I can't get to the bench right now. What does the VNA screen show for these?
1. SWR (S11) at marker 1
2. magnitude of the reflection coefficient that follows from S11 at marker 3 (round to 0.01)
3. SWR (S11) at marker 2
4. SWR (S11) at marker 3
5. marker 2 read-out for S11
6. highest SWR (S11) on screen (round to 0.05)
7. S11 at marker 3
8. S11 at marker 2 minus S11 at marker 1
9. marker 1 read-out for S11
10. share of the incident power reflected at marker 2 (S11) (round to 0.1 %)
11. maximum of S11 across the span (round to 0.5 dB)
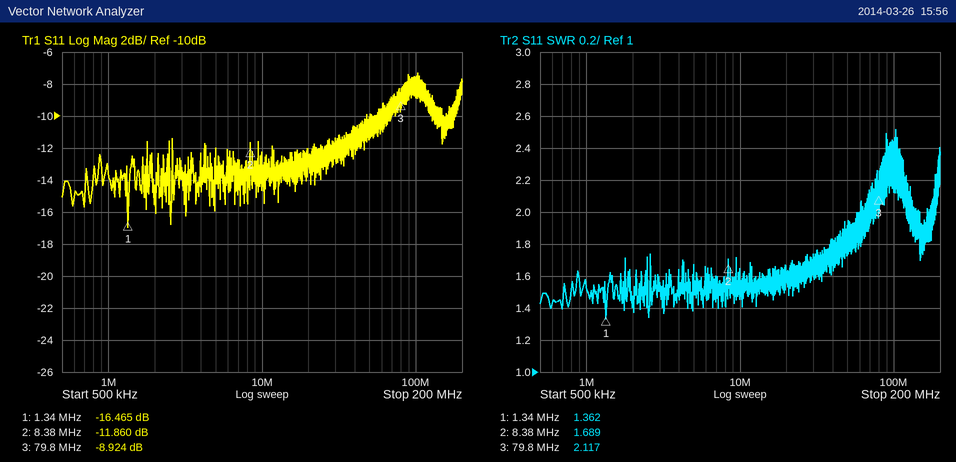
1.362
0.36
1.689
2.117
-11.860 dB
2.50
-8.924 dB
4.605 dB
-16.465 dB
6.5 %
-7.5 dB
